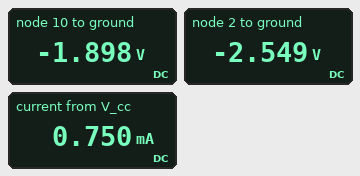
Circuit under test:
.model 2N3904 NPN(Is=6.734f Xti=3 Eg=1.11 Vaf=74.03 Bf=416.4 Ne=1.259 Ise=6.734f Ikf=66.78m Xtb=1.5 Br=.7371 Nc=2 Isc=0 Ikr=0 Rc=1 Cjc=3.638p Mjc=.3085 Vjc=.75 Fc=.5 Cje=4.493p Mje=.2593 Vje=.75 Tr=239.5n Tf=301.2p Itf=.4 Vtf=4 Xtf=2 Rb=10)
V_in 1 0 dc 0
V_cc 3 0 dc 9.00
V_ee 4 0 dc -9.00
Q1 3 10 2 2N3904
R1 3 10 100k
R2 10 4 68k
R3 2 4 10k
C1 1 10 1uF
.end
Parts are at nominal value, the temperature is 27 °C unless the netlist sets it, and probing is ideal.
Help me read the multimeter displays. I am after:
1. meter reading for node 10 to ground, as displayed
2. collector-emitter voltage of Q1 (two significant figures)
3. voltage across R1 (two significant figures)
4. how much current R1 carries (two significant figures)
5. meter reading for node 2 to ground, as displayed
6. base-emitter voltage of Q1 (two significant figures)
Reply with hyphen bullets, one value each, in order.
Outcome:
- -1.898 V
- 12 V
- 11 V
- 110 µA
- -2.549 V
- 650 mV
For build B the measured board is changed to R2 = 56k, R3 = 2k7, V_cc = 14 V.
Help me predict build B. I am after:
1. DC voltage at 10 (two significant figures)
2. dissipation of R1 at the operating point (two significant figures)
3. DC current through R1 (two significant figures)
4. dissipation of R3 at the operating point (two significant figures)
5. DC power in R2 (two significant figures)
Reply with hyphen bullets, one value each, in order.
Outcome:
- -1.3 V
- 2.3 mW
- 150 µA
- 18 mW
- 1.1 mW
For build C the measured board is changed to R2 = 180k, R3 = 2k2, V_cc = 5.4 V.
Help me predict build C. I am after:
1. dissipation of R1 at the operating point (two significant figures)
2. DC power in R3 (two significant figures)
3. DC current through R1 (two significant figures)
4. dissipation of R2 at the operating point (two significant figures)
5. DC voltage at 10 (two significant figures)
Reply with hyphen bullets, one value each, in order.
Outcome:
- 410 µW
- 24 mW
- 64 µA
- 350 µW
- -1.0 V
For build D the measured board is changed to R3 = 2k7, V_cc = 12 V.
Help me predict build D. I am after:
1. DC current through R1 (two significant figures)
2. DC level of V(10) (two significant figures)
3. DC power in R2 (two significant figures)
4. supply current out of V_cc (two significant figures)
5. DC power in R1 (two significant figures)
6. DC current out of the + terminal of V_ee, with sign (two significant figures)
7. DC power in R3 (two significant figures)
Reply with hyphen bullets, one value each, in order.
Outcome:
- 130 µA
- -1.1 V
- 910 µW
- 2.8 mA
- 1.7 mW
- -2.8 mA
- 19 mW
